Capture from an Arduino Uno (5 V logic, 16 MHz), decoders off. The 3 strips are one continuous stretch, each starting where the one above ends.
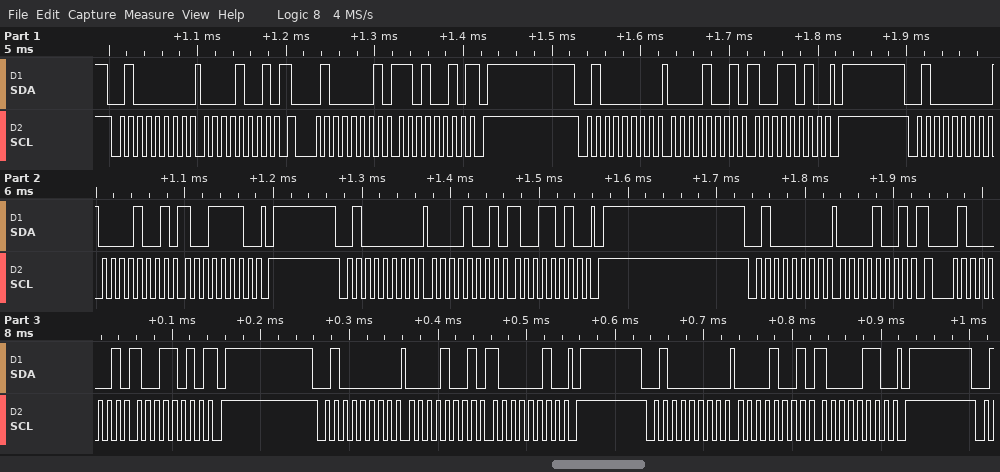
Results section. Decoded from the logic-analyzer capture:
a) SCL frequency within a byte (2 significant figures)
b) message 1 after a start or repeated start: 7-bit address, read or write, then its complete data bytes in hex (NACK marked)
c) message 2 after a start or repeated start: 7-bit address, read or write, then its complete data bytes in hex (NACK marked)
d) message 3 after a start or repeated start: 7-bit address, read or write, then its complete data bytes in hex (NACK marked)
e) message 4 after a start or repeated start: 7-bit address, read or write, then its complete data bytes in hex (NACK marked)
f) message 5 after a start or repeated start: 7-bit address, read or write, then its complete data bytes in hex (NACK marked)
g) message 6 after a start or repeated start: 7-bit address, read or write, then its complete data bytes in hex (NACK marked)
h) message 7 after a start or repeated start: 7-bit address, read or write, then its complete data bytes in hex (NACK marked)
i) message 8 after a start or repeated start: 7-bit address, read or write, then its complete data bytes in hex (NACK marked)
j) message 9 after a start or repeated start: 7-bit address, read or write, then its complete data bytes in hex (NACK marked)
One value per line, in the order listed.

100 kHz
0x20 write: 09
0x20 read: D2 NACK
0x20 write: 09 9A
0x20 write: 09 9E
0x20 write: 09 9A
0x20 write: 09
0x20 read: 9A NACK
0x20 write: 09 82
0x20 write: 09 86
